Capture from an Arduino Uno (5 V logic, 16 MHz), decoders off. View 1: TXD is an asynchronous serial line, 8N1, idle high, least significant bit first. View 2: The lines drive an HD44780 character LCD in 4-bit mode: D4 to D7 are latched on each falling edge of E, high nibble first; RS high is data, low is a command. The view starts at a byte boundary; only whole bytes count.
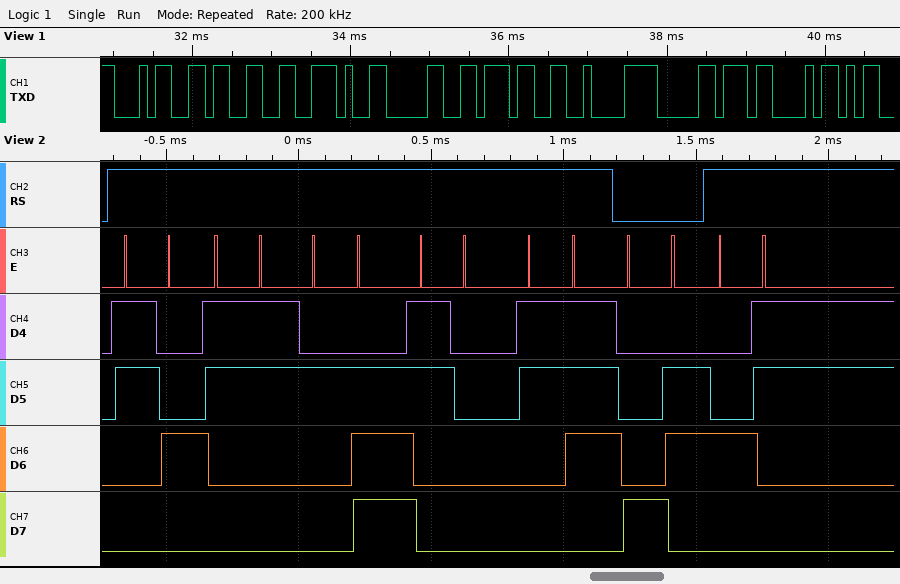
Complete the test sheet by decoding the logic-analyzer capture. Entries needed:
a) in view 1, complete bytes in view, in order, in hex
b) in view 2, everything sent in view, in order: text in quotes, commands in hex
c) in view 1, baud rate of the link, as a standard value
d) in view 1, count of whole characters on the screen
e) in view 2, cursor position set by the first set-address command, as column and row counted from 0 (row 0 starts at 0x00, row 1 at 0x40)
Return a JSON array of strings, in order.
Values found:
["0x34 0x33 0x2E 0x30 0x37 0xC2 0xB0 0x43", "\"43.07\" 0x86 \"C\"", "9600 baud", "8", "column 6, row 0"]
